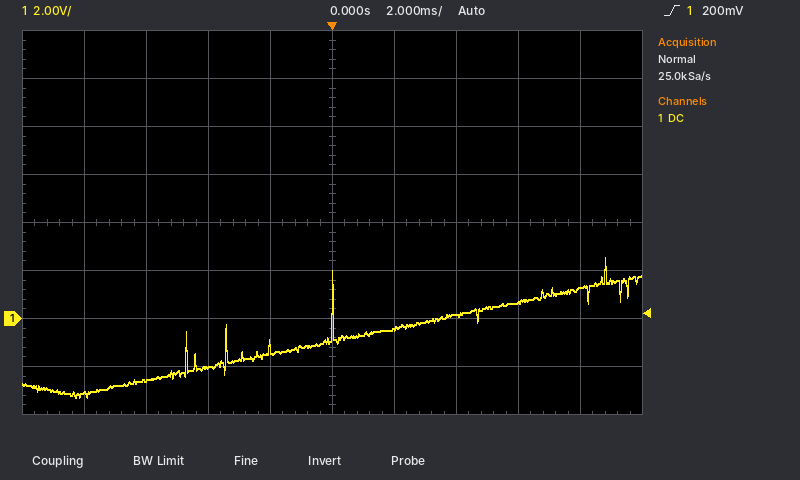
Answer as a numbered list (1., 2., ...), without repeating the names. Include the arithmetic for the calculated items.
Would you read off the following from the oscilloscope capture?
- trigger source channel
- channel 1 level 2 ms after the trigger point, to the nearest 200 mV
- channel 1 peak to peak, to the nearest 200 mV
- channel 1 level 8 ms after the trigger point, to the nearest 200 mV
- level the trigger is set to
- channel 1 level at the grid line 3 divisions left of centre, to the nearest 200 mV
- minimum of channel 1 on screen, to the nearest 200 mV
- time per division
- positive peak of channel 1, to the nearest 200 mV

1. channel 1
2. -400 mV
3. 2.6 V − (-3.2 V) = 5.8 V
4. 1.2 V
5. 200 mV
6. -2.6 V
7. -3.2 V
8. 2 ms
9. 2.6 V
